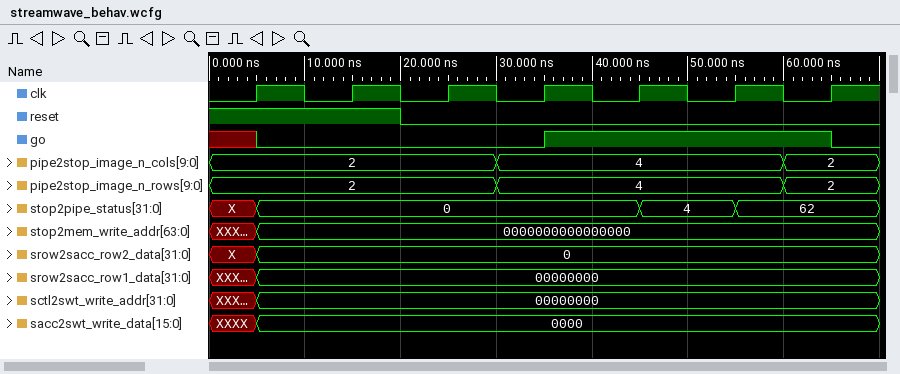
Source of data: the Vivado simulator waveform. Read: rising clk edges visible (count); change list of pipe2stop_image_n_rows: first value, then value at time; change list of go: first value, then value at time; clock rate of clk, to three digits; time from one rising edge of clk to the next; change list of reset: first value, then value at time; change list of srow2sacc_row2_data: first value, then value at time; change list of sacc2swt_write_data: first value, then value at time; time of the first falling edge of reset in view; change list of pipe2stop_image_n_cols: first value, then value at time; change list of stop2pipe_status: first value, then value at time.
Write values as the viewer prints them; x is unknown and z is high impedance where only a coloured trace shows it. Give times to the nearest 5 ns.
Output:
7
2, 4 at 30 ns, 2 at 60 ns
x, 0 at 5 ns, 1 at 35 ns, 0 at 65 ns
100 MHz
10 ns
1, 0 at 20 ns
X, 0 at 5 ns
XXXX, 0000 at 5 ns
20 ns
2, 4 at 30 ns, 2 at 60 ns
X, 0 at 5 ns, 4 at 45 ns, 62 at 55 ns
